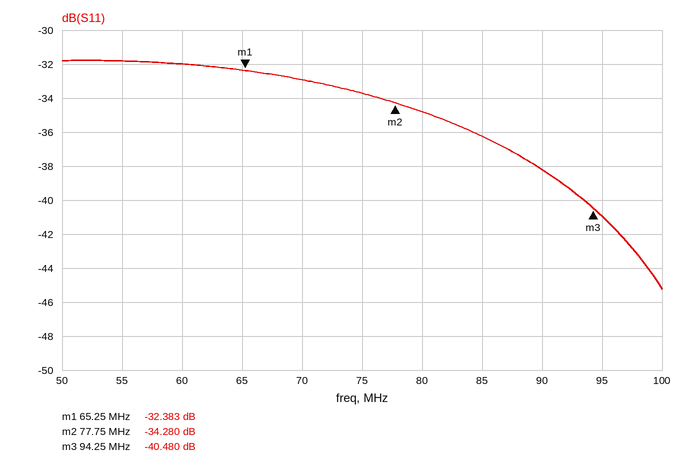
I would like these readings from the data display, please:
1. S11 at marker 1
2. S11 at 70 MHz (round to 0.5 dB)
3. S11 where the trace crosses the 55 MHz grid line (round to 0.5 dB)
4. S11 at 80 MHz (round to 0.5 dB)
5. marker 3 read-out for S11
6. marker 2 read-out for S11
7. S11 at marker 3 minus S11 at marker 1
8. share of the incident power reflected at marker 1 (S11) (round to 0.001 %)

-32.383 dB
-33.0 dB
-32.0 dB
-35.0 dB
-40.480 dB
-34.280 dB
-8.097 dB
0.058 %
